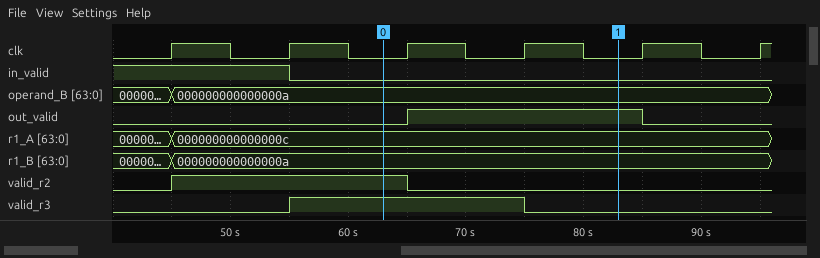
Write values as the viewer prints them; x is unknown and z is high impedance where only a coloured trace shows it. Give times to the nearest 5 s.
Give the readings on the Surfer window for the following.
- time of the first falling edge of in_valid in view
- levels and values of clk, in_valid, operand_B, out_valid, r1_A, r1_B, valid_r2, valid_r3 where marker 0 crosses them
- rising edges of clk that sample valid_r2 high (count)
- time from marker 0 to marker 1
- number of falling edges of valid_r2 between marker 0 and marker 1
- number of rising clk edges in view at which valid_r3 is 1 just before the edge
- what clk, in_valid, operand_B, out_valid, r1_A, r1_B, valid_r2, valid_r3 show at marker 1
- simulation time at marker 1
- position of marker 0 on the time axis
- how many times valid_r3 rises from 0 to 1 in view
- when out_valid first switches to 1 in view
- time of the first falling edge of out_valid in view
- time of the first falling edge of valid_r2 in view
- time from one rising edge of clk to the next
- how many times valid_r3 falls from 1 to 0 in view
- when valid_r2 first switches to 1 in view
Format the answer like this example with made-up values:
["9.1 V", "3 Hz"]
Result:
["55 s", "clk=0, in_valid=0, operand_B=000000000000000a, out_valid=0, r1_A=000000000000000c, r1_B=000000000000000a, valid_r2=1, valid_r3=1", "2", "20 s", "1", "2", "clk=0, in_valid=0, operand_B=000000000000000a, out_valid=1, r1_A=000000000000000c, r1_B=000000000000000a, valid_r2=0, valid_r3=0", "85 s", "65 s", "1", "65 s", "85 s", "65 s", "10 s", "1", "45 s"]
